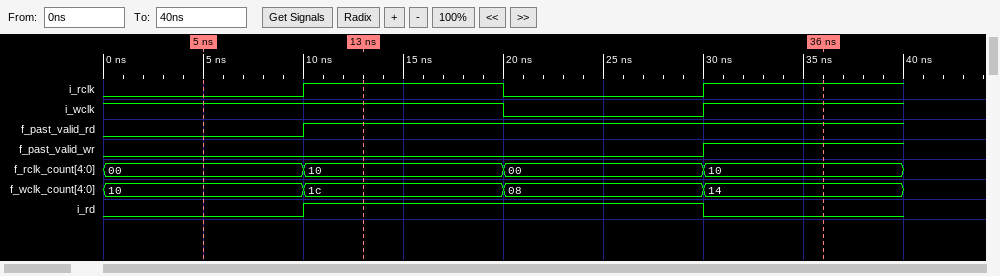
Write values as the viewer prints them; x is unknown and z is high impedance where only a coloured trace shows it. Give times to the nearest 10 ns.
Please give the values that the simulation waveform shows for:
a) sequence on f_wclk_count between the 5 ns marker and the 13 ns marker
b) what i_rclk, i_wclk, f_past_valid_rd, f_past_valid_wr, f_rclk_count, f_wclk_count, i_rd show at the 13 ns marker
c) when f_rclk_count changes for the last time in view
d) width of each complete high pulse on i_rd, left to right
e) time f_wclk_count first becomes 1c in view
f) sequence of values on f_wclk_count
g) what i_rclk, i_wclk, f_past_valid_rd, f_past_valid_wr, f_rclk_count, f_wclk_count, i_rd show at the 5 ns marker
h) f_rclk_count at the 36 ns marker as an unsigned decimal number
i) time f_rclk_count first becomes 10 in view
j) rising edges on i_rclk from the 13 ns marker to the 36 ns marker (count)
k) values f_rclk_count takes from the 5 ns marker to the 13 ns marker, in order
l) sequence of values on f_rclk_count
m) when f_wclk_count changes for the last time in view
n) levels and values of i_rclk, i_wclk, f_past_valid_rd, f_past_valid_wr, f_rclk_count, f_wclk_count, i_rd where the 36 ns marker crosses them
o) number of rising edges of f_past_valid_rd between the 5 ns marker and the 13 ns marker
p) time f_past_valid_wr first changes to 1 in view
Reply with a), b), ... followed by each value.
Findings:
a) 10, 1c
b) i_rclk=1, i_wclk=1, f_past_valid_rd=1, f_past_valid_wr=0, f_rclk_count=10, f_wclk_count=1c, i_rd=1
c) 30 ns
d) 20 ns
e) 10 ns
f) 10, 1c, 08, 14
g) i_rclk=0, i_wclk=1, f_past_valid_rd=0, f_past_valid_wr=0, f_rclk_count=00, f_wclk_count=10, i_rd=0
h) 16
i) 10 ns
j) 1
k) 00, 10
l) 00, 10, 00, 10
m) 30 ns
n) i_rclk=1, i_wclk=1, f_past_valid_rd=1, f_past_valid_wr=1, f_rclk_count=10, f_wclk_count=14, i_rd=0
o) 1
p) 30 ns
